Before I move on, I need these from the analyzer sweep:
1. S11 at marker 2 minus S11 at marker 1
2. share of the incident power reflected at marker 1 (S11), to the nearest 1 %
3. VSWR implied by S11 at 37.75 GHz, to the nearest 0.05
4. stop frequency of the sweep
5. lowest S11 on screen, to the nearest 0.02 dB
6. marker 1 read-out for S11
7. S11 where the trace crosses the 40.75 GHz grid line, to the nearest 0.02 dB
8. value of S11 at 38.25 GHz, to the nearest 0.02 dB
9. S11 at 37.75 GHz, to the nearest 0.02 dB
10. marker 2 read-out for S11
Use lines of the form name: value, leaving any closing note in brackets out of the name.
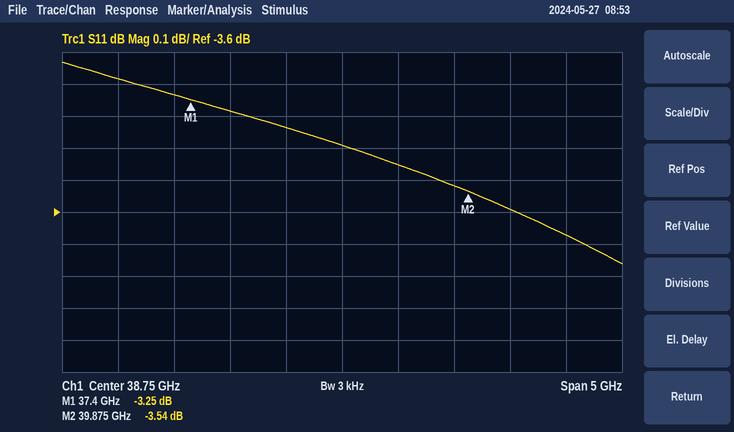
S11 at marker 2 minus S11 at marker 1: -0.29 dB
share of the incident power reflected at marker 1 (S11), to the nearest 1 %: 47 %
VSWR implied by S11 at 37.75 GHz, to the nearest 0.05: 5.35
stop frequency of the sweep: 41.25 GHz
lowest S11 on screen, to the nearest 0.02 dB: -3.76 dB
marker 1 read-out for S11: -3.25 dB
S11 where the trace crosses the 40.75 GHz grid line, to the nearest 0.02 dB: -3.68 dB
value of S11 at 38.25 GHz, to the nearest 0.02 dB: -3.34 dB
S11 at 37.75 GHz, to the nearest 0.02 dB: -3.28 dB
marker 2 read-out for S11: -3.54 dB
